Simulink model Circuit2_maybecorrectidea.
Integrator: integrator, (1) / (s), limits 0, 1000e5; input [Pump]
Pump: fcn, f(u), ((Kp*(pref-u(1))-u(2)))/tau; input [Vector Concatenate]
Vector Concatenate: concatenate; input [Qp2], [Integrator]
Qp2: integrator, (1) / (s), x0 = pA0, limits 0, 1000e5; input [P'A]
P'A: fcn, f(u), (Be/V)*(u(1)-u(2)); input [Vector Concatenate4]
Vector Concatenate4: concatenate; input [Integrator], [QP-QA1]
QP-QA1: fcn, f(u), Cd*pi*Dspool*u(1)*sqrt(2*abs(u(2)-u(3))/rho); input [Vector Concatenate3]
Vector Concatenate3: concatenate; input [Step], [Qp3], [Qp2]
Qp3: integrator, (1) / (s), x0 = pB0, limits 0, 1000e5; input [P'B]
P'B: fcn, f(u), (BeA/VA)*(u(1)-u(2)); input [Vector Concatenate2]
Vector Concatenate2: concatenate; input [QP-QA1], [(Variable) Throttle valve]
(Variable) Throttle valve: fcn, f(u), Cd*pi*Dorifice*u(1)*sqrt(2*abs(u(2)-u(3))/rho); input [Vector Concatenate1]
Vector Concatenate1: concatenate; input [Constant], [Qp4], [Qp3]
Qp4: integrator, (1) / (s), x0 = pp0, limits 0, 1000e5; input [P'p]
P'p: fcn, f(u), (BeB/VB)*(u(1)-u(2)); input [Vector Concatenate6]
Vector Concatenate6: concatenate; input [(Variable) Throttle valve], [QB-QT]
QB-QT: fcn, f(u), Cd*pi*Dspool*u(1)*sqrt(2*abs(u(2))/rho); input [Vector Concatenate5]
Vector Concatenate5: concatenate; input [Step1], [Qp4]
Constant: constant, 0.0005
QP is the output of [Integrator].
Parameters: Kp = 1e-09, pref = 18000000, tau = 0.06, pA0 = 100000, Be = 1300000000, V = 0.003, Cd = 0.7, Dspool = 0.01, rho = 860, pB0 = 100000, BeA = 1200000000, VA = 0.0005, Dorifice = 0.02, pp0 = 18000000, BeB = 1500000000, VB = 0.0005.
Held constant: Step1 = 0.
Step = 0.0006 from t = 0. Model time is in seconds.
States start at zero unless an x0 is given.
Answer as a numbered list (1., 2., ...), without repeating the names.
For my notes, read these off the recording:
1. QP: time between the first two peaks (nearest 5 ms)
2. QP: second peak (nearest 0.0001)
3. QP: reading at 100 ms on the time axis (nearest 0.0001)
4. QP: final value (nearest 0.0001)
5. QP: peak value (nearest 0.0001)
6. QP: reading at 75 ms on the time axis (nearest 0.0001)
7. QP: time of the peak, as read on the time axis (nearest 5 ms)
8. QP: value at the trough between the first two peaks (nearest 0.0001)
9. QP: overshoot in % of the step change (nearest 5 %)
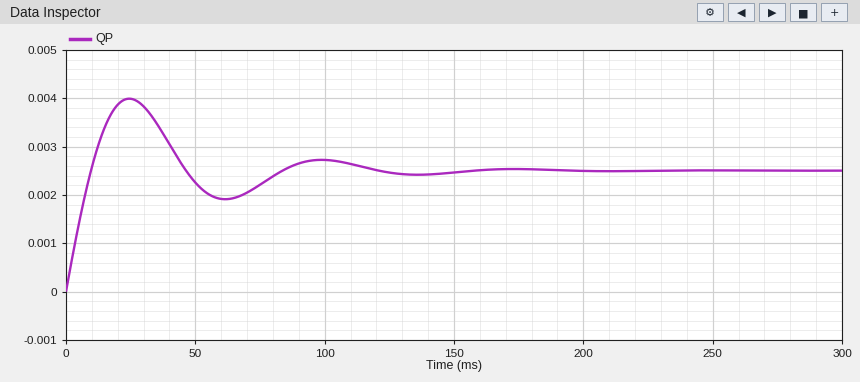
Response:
1. 75 ms
2. 0.0027
3. 0.0027
4. 0.0025
5. 0.0040
6. 0.0022
7. 25 ms
8. 0.0019
9. 60 %
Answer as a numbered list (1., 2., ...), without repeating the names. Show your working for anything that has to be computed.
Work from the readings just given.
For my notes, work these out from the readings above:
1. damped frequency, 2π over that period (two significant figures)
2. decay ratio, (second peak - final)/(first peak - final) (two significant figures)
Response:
1. 2π / 75 = 0.084 rad/ms
2. (0.0027 - 0.0025) / (0.004 - 0.0025) = 0.13
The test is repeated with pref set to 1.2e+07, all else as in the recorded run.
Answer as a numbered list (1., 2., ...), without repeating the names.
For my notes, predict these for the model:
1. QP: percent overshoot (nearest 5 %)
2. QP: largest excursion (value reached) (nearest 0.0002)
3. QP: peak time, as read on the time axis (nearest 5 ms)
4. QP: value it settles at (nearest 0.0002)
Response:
1. 40 %
2. 0.0028
3. 25 ms
4. 0.0020
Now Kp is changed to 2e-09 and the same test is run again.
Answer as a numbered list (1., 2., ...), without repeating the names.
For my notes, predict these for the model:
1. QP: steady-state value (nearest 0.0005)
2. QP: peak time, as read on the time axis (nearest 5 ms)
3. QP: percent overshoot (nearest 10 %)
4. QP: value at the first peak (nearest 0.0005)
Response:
1. 0.0025
2. 15 ms
3. 110 %
4. 0.0055
